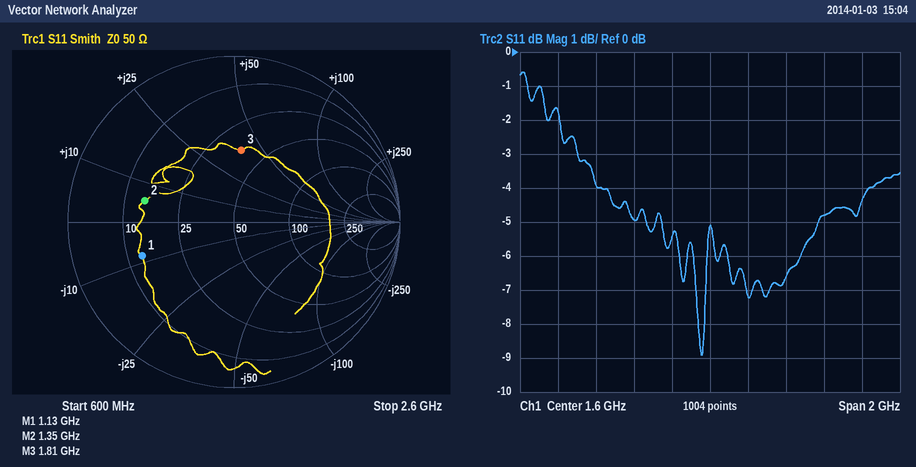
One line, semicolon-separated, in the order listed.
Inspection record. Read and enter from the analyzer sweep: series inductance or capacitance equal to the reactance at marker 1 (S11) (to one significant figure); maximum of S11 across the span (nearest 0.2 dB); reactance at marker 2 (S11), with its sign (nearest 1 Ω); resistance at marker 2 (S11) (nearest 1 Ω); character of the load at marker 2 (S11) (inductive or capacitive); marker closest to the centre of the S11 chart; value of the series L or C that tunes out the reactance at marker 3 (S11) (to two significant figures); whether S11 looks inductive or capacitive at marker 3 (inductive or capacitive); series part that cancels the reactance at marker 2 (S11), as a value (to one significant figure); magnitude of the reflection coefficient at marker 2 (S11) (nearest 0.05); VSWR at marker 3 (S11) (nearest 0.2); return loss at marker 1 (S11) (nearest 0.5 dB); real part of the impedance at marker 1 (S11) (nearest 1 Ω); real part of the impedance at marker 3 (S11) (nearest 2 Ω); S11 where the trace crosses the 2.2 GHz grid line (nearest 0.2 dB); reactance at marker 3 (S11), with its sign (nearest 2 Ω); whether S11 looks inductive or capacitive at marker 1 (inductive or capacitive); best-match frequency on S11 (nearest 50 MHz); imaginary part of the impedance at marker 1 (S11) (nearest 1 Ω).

20 pF; -0.6 dB; +5 Ω; 15 Ω; inductive; marker 3; 2.2 pF; inductive; 20 pF; 0.55; 2.6; 4.5 dB; 13 Ω; 36 Ω; -4.8 dB; +40 Ω; capacitive; 1.55 GHz; -8 Ω
